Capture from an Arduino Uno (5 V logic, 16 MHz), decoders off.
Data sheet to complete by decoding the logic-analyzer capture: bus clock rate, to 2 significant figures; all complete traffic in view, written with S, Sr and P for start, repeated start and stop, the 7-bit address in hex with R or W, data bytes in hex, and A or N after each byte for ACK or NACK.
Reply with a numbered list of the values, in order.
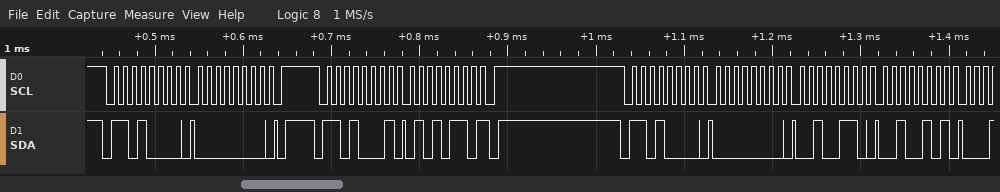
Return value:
1. 100 kHz
2. S 68W A 00 A P S 68R A 56 N P S 68W A 00 A 26 A 25 A
